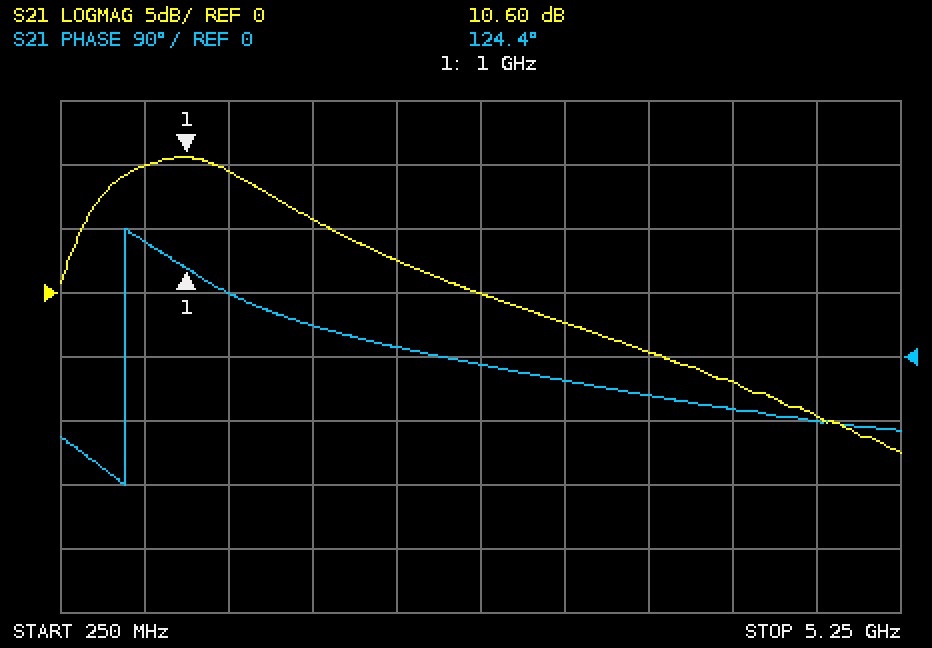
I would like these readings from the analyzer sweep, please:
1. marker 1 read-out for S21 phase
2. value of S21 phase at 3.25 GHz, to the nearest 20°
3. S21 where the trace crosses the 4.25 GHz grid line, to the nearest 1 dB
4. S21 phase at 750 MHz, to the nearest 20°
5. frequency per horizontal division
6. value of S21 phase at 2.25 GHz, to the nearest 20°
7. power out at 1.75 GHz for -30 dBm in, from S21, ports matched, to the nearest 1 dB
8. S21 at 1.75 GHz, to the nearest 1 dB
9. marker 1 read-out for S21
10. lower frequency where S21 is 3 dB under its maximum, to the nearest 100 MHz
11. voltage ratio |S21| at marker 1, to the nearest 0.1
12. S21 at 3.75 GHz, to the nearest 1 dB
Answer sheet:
124.4°
-40°
-7 dB
160°
500 MHz
20°
-24 dBm
6 dB
10.60 dB
500 MHz
3.4
-5 dB
